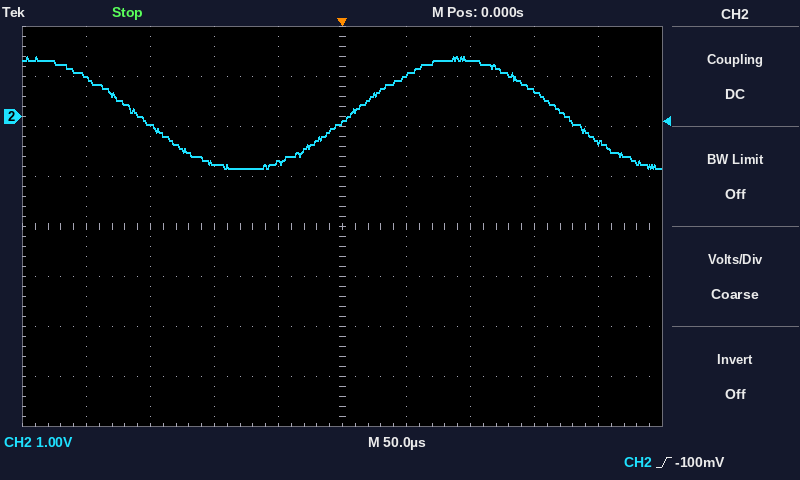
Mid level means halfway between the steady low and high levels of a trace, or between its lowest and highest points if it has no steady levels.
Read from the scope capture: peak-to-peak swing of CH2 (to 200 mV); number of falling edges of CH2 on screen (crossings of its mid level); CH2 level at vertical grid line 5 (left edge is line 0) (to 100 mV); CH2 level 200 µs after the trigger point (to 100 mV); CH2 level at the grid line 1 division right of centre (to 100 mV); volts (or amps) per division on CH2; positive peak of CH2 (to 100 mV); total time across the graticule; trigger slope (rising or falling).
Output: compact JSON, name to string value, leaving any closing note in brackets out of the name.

{"peak-to-peak swing of CH2": "2.2 V", "number of falling edges of CH2 on screen": "2", "CH2 level at vertical grid line 5 (left edge is line 0)": "-100 mV", "CH2 level 200 µs after the trigger point": "-500 mV", "CH2 level at the grid line 1 division right of centre": "800 mV", "volts (or amps) per division on CH2": "1 V", "positive peak of CH2": "1.2 V", "total time across the graticule": "500 µs", "trigger slope": "rising"}
